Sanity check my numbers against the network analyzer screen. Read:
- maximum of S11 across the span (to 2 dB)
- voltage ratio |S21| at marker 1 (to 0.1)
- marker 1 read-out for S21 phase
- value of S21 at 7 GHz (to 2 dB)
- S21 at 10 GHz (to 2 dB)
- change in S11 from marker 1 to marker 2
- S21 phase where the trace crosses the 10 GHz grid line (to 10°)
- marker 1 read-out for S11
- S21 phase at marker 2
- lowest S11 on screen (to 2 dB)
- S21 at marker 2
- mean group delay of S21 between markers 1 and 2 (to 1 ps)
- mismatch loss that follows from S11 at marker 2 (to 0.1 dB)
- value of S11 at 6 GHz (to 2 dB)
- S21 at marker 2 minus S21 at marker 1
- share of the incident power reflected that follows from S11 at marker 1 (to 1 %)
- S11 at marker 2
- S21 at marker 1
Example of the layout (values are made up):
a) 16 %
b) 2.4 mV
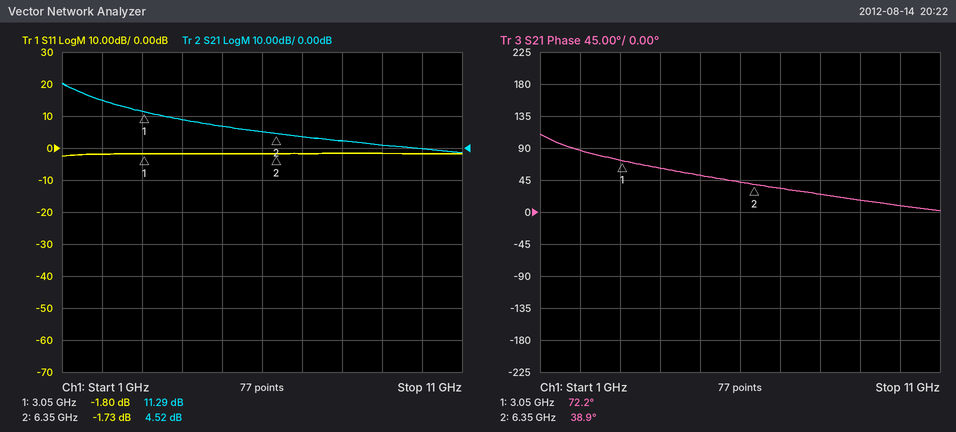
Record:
a) -2 dB
b) 3.7
c) 72.2°
d) 4 dB
e) 0 dB
f) 0.07 dB
g) 10°
h) -1.80 dB
i) 38.9°
j) -2 dB
k) 4.52 dB
l) 28 ps
m) 4.8 dB
n) -2 dB
o) -6.77 dB
p) 66 %
q) -1.73 dB
r) 11.29 dB
